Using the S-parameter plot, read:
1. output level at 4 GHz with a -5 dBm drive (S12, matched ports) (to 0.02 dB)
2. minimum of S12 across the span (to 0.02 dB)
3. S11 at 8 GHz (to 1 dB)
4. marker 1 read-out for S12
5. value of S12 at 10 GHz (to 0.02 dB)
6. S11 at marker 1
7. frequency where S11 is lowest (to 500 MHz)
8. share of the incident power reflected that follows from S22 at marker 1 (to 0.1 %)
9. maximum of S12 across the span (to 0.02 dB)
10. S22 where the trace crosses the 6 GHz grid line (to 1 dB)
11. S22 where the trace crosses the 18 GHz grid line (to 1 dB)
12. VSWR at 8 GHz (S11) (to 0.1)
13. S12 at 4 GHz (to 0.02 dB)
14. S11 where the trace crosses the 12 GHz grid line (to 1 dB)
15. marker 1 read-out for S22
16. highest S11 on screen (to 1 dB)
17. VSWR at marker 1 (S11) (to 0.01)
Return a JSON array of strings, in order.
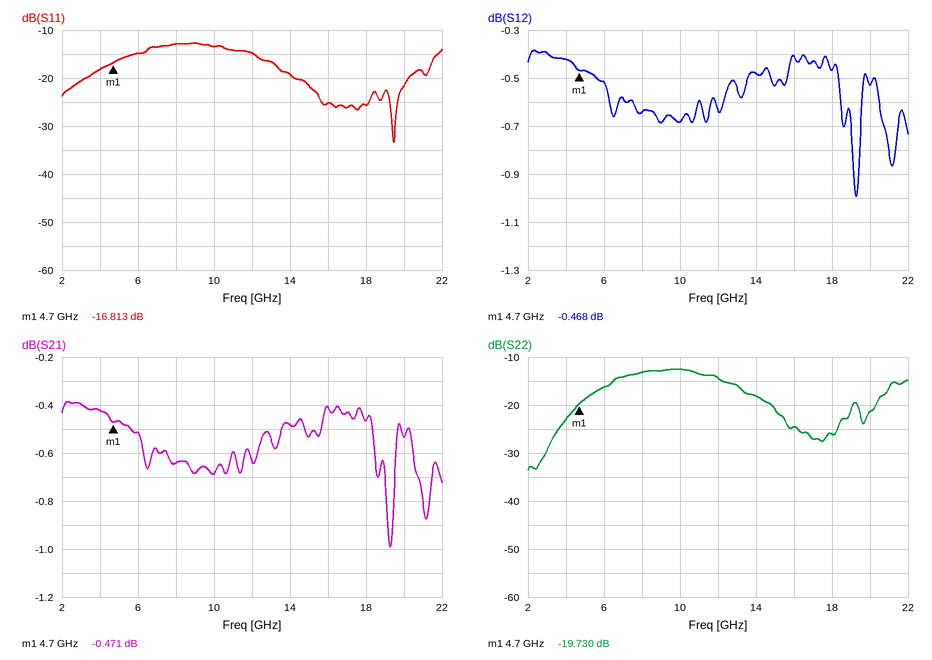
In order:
["-5.42 dBm", "-1.00 dB", "-13 dB", "-0.468 dB", "-0.68 dB", "-16.813 dB", "19.5 GHz", "1.1 %", "-0.38 dB", "-16 dB", "-26 dB", "1.6", "-0.42 dB", "-15 dB", "-19.730 dB", "-13 dB", "1.34"]
